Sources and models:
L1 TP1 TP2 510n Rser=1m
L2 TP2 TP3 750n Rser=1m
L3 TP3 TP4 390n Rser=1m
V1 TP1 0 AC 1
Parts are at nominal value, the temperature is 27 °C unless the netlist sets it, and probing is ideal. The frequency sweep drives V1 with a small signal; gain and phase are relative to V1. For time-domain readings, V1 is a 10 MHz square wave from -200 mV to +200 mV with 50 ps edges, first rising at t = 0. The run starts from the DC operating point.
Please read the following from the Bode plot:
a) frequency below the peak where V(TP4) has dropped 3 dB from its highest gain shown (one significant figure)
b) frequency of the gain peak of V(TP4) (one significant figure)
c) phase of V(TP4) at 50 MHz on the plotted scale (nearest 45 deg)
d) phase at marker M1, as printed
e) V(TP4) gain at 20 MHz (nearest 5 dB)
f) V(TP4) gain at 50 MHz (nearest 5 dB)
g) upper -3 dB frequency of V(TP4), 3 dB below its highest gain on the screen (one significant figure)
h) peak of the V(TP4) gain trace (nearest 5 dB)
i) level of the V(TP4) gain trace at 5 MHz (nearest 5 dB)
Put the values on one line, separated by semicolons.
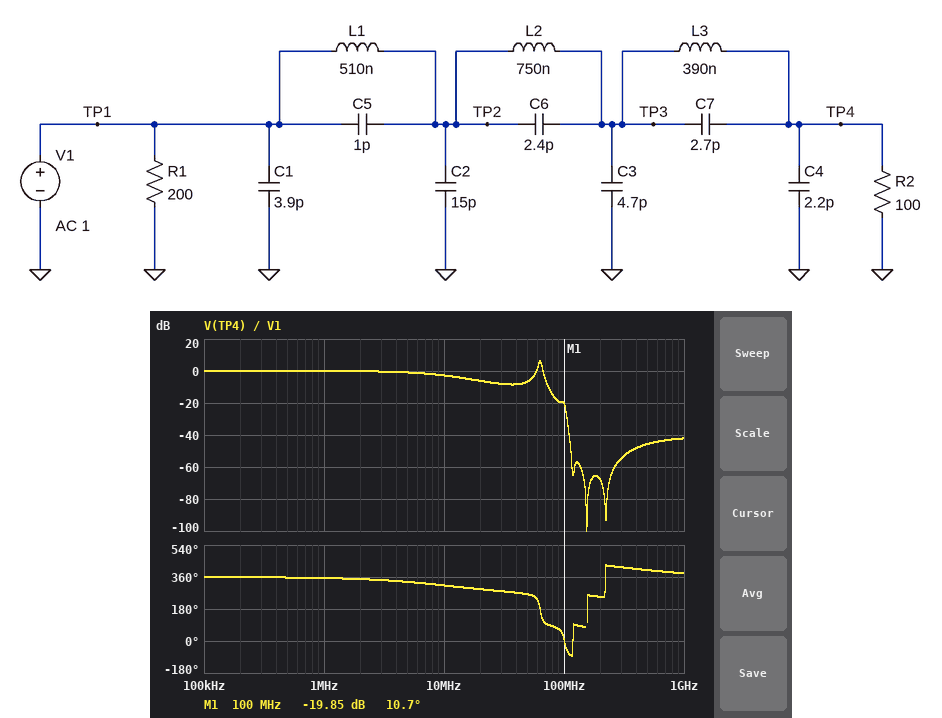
60 MHz; 60 MHz; 270 deg; 10.7 deg; -5 dB; -5 dB; 70 MHz; 5 dB; 0 dB
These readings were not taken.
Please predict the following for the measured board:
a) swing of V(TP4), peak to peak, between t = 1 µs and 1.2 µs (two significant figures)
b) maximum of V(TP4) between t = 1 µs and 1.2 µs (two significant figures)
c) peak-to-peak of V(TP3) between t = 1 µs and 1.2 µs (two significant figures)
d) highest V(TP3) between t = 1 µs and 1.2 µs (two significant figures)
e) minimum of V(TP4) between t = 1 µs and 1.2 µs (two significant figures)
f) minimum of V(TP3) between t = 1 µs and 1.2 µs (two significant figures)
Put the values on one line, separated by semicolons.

400 mV; 200 mV; 460 mV; 230 mV; -200 mV; -230 mV
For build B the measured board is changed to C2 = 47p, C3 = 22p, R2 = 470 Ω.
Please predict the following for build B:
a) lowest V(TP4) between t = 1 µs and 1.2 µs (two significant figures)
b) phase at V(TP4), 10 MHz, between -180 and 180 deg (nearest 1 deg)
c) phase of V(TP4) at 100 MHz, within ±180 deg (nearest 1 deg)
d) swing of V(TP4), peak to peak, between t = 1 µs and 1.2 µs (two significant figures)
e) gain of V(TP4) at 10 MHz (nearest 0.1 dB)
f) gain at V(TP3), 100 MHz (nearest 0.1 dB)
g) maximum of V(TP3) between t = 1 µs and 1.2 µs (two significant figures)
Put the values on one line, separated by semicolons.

-560 mV; -14 deg; -54 deg; 1.1 V; 1.8 dB; -46.4 dB; 550 mV
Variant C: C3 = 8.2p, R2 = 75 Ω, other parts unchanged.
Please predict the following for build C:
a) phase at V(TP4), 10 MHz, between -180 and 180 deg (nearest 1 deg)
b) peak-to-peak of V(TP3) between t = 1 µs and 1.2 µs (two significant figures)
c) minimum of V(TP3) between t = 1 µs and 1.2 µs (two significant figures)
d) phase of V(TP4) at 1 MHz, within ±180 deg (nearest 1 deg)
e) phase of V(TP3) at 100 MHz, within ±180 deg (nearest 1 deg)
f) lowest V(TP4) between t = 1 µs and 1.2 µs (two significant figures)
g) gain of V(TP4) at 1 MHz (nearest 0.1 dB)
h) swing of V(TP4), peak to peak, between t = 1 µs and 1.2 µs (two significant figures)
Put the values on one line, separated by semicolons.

-56 deg; 400 mV; -200 mV; -8 deg; 11 deg; -170 mV; -0.1 dB; 350 mV
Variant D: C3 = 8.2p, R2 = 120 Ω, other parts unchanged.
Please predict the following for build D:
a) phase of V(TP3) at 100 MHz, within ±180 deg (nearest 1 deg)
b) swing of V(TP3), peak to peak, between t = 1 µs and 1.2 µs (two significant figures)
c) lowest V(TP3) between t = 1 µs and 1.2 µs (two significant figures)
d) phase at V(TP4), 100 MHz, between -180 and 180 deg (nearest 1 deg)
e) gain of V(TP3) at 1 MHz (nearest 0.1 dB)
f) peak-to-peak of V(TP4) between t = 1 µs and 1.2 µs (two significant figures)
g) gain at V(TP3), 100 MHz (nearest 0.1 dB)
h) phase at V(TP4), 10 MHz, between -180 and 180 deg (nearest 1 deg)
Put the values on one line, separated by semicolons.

17 deg; 470 mV; -240 mV; -66 deg; 0 dB; 420 mV; -19.5 dB; -43 deg
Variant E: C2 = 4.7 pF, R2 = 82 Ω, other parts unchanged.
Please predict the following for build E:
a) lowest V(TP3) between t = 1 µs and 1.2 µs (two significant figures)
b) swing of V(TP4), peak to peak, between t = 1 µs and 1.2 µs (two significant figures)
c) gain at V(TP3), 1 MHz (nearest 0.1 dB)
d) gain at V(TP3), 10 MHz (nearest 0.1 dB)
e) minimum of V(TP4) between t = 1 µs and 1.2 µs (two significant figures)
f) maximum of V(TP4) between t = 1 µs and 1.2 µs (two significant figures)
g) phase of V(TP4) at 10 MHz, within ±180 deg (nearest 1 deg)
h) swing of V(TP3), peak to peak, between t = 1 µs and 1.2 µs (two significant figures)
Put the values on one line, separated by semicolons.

-260 mV; 370 mV; -0.1 dB; -3.6 dB; -190 mV; 190 mV; -53 deg; 510 mV
